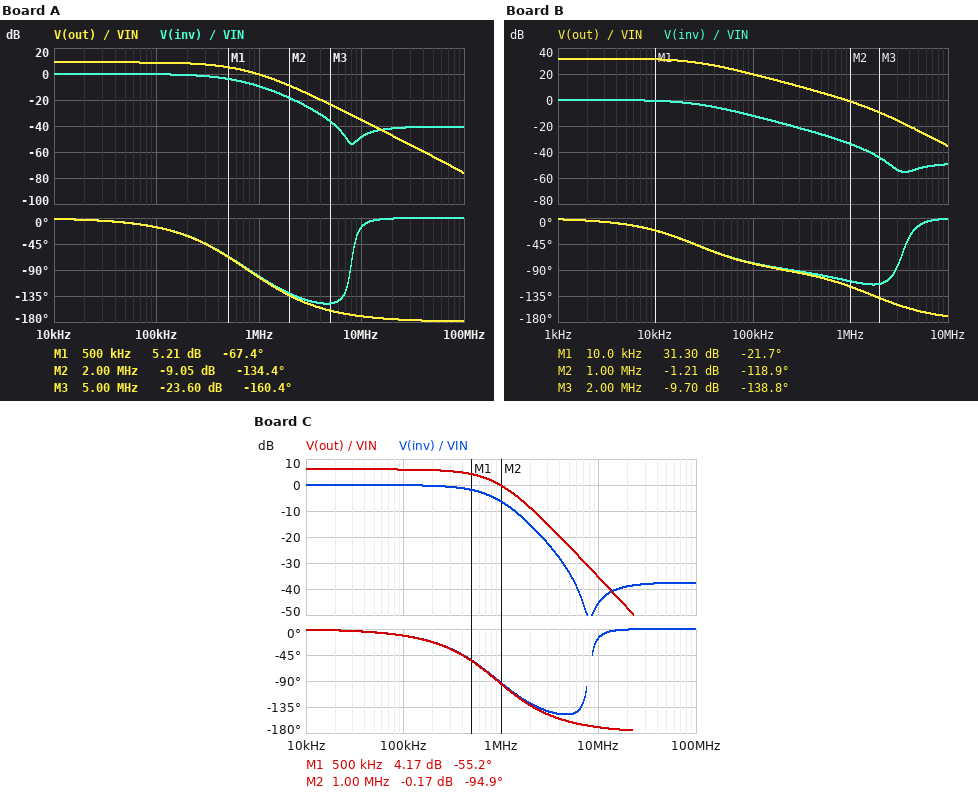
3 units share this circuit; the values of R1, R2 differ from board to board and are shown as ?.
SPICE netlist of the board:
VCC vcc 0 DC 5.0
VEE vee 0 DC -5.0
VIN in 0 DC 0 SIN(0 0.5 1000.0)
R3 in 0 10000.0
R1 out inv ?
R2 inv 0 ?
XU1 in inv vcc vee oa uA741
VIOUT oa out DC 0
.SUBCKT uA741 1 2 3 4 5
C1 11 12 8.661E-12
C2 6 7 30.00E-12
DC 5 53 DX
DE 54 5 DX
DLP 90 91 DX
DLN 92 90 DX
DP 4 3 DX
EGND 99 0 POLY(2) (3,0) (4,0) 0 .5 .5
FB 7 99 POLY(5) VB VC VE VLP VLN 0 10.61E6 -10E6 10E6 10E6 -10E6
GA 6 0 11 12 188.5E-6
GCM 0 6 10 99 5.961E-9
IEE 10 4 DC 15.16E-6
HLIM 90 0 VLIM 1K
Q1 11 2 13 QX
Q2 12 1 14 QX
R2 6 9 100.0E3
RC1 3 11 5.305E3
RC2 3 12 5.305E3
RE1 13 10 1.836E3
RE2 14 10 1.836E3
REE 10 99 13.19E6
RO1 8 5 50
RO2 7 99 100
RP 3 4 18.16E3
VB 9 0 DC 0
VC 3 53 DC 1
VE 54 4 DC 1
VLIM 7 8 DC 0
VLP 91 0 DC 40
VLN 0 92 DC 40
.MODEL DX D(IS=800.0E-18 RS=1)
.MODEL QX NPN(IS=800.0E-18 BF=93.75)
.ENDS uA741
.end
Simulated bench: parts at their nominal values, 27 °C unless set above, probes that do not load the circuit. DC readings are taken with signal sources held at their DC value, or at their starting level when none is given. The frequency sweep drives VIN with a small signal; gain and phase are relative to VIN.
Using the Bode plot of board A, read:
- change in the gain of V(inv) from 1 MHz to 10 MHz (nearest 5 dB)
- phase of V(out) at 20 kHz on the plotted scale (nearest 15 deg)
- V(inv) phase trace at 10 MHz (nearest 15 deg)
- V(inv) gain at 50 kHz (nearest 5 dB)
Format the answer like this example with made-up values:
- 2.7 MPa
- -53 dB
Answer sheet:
- -40 dB
- 0 deg
- -15 deg
- 0 dB
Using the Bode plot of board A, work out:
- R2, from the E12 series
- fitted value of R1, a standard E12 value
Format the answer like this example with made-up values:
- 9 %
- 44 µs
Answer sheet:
- 15 kΩ
- 27 kΩ
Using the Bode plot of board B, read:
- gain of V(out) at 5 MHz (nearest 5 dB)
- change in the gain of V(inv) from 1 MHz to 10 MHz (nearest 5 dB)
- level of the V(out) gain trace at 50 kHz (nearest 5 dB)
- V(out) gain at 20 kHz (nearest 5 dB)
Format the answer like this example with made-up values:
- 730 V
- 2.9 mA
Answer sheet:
- -25 dB
- -15 dB
- 25 dB
- 30 dB
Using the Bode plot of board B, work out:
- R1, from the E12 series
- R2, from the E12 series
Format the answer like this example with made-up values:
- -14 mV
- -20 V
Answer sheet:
- 150 kΩ
- 3.9 kΩ
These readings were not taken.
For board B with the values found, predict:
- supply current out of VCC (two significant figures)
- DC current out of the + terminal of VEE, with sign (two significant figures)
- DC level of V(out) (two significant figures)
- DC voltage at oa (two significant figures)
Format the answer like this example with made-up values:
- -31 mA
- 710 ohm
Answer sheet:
- 570 µA
- -570 µA
- 13 mV
- 13 mV
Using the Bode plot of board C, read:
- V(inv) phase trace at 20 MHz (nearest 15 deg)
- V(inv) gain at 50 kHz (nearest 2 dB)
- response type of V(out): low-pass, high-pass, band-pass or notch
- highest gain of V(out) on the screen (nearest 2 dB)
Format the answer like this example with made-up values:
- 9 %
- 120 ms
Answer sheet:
- 0 deg
- 0 dB
- low-pass
- 6 dB
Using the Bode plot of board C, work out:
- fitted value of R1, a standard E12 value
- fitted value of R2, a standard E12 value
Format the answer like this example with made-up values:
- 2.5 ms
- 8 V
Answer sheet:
- 27 kΩ
- 27 kΩ
